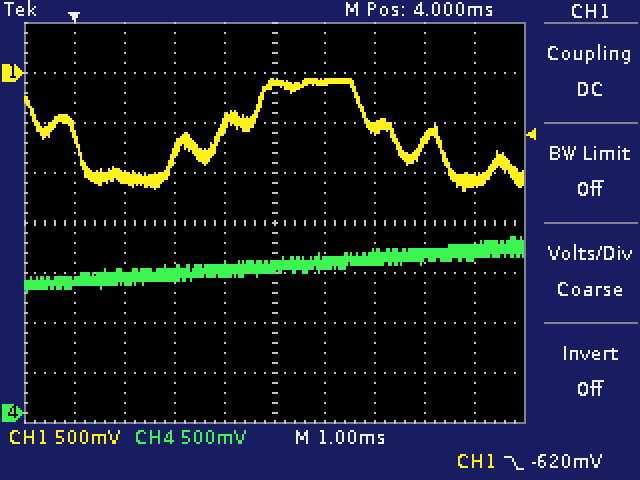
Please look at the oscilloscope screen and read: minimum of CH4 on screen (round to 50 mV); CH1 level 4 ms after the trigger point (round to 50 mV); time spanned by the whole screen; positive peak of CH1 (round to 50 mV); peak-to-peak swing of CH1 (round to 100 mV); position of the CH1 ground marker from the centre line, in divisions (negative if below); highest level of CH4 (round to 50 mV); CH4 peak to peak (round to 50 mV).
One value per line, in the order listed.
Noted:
1.20 V
-100 mV
10 ms
-50 mV
1.10 V
+3.0 div
1.75 V
550 mV
